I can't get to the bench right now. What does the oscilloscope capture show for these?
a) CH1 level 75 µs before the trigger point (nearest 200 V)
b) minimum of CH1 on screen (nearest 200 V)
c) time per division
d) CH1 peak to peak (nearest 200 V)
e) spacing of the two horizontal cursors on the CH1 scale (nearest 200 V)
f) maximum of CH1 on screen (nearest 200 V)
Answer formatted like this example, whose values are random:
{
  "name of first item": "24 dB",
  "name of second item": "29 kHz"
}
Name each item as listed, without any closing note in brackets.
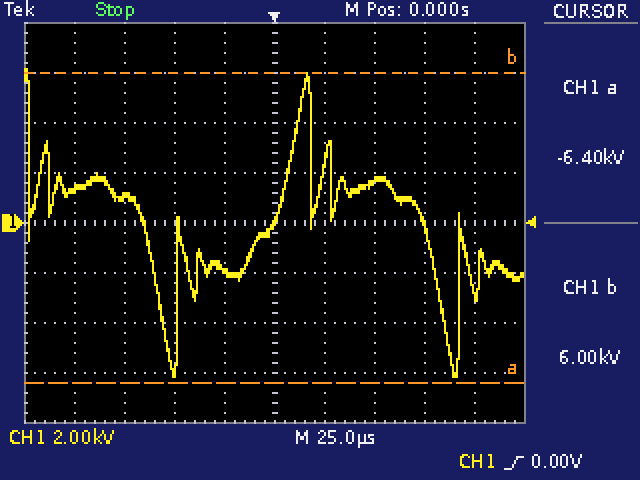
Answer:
{
  "CH1 level 75 µs before the trigger point": "1.0 kV",
  "minimum of CH1 on screen": "-6.2 kV",
  "time per division": "25 µs",
  "CH1 peak to peak": "12.4 kV",
  "spacing of the two horizontal cursors on the CH1 scale": "12.4 kV",
  "maximum of CH1 on screen": "6.2 kV"
}
